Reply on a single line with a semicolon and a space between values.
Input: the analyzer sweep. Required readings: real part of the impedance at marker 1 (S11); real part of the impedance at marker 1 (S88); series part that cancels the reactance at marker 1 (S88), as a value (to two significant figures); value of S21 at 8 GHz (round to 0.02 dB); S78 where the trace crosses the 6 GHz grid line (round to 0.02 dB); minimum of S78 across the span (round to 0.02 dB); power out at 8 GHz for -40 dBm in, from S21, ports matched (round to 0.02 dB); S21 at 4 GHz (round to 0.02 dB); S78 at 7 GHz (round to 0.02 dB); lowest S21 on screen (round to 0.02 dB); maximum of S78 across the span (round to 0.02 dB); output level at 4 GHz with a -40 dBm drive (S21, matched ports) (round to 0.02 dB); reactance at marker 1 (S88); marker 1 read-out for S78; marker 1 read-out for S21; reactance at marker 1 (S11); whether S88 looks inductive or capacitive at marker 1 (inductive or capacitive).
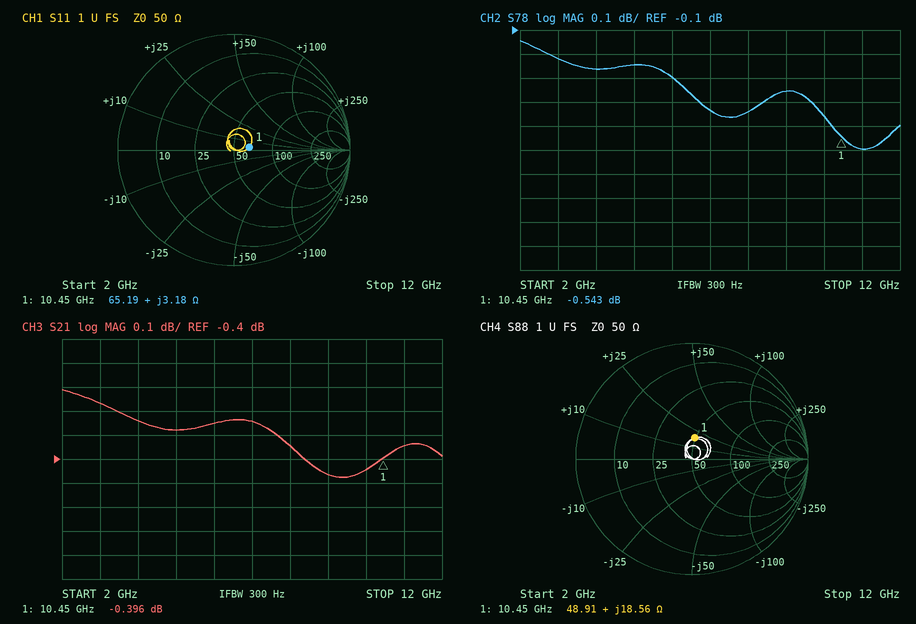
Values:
65.19 Ω; 48.91 Ω; 820 fF; -0.34 dB; -0.30 dB; -0.60 dB; -40.34 dBm; -0.24 dB; -0.44 dB; -0.48 dB; -0.14 dB; -40.24 dBm; +18.56 Ω; -0.543 dB; -0.396 dB; +3.18 Ω; inductive
